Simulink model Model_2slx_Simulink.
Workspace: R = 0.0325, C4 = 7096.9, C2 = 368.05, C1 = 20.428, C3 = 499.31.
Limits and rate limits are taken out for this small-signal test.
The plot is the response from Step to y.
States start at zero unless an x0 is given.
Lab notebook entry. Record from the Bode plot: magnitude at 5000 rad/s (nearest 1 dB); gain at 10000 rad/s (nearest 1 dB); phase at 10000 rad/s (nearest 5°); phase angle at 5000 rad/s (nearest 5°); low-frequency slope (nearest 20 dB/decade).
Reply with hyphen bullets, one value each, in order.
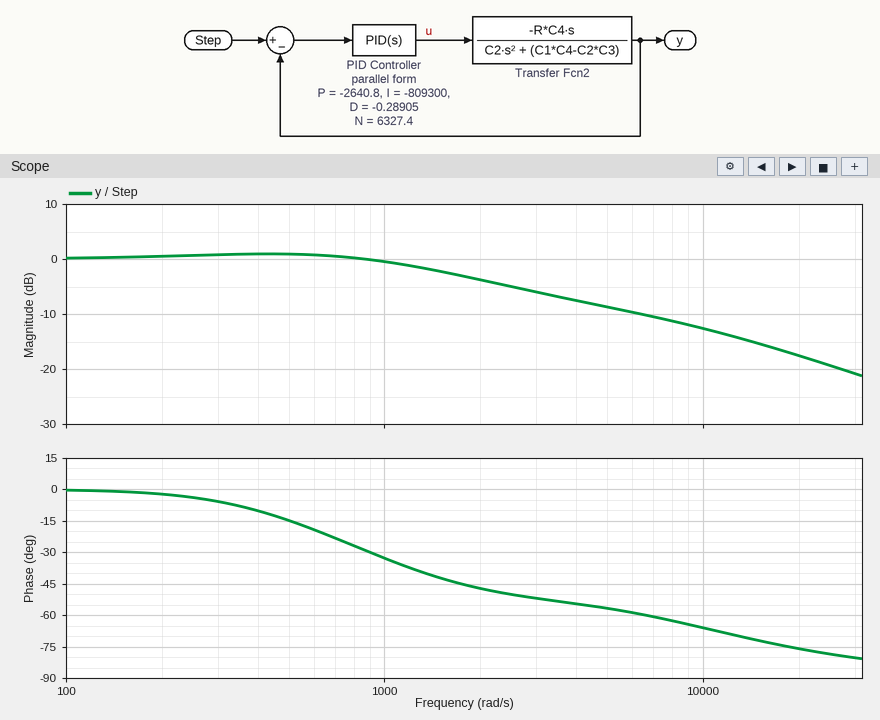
- -9 dB
- -13 dB
- -65°
- -55°
- 0 dB/decade
